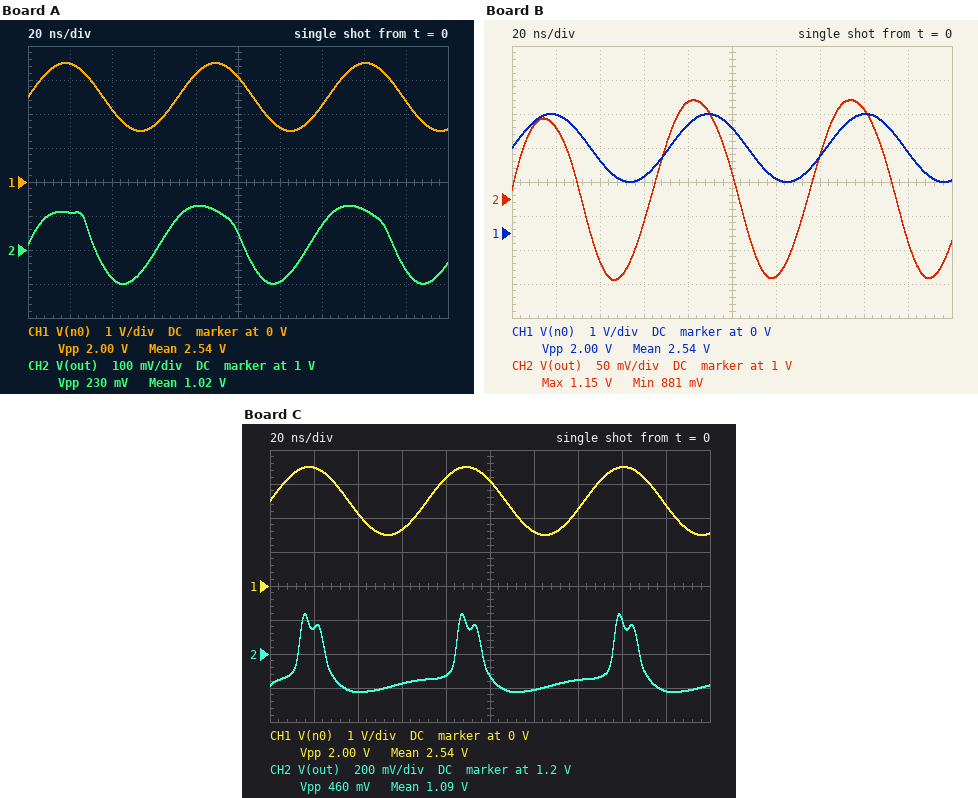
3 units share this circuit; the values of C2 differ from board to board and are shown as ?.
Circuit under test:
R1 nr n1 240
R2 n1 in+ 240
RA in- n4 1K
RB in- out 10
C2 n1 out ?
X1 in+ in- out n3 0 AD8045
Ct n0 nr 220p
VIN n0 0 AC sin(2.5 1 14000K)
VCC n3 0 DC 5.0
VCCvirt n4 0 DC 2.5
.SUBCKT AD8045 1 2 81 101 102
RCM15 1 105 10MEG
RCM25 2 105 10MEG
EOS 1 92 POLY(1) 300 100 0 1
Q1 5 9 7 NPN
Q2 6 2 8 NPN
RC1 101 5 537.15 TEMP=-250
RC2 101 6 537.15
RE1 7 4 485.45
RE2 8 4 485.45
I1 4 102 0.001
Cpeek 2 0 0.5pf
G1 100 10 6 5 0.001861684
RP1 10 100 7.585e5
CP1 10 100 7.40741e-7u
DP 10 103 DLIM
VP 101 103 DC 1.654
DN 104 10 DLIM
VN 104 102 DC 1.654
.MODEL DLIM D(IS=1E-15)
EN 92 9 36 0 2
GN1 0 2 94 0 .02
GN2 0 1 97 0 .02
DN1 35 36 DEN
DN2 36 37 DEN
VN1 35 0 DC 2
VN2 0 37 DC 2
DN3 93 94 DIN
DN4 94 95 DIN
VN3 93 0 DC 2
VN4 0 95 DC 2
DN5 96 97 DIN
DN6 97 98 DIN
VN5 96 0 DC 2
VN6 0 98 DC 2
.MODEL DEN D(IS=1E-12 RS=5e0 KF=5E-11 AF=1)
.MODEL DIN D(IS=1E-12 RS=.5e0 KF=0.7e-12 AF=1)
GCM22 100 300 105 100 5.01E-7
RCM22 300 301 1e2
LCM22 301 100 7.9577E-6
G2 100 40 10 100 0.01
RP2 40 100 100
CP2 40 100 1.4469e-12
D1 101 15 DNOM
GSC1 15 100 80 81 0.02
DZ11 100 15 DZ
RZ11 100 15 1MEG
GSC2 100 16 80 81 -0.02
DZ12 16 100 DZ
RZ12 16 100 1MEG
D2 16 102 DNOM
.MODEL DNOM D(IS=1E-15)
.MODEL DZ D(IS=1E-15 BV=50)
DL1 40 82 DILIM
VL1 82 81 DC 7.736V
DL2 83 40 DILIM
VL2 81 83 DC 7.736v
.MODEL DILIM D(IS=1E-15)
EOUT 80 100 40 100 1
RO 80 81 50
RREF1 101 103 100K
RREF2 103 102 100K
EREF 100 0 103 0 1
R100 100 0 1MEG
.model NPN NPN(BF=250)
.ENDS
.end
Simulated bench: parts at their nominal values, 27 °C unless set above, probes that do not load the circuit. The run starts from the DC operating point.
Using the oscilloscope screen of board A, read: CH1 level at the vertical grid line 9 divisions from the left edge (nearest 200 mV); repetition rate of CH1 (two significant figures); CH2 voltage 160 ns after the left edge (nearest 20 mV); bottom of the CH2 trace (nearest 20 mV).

2.4 V
14 MHz
1.12 V
900 mV
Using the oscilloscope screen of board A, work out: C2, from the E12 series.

47 pF
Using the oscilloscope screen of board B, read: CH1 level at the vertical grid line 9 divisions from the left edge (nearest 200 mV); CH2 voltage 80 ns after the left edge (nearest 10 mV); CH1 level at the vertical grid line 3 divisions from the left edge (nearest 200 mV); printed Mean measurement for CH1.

2.4 V
1.14 V
1.6 V
2.54 V
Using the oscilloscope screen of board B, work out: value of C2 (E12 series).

68 pF
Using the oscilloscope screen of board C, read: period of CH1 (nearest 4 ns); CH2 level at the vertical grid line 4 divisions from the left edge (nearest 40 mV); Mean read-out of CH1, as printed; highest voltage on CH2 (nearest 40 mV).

72 ns
1.08 V
2.54 V
1.44 V
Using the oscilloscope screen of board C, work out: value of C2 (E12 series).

10 pF
